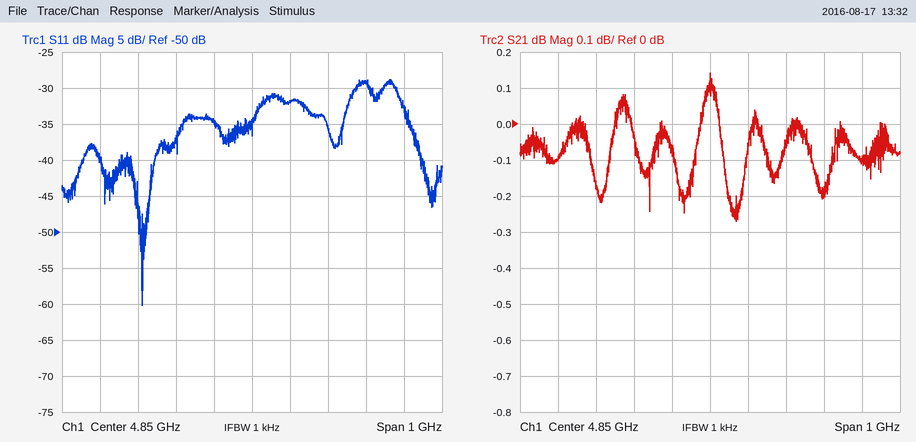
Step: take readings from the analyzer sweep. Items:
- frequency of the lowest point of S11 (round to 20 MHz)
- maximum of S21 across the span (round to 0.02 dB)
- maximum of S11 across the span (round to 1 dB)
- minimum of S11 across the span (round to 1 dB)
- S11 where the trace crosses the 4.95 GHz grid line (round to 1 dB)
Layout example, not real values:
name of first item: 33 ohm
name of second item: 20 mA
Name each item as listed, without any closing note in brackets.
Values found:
frequency of the lowest point of S11: 4.56 GHz
maximum of S21 across the span: 0.14 dB
maximum of S11 across the span: -29 dB
minimum of S11 across the span: -60 dB
S11 where the trace crosses the 4.95 GHz grid line: -32 dB
